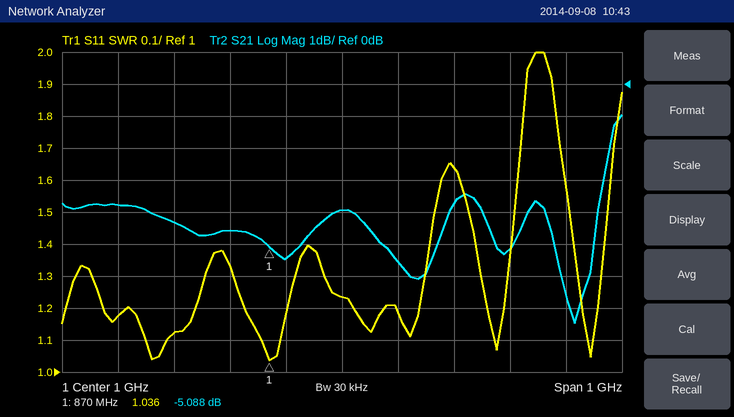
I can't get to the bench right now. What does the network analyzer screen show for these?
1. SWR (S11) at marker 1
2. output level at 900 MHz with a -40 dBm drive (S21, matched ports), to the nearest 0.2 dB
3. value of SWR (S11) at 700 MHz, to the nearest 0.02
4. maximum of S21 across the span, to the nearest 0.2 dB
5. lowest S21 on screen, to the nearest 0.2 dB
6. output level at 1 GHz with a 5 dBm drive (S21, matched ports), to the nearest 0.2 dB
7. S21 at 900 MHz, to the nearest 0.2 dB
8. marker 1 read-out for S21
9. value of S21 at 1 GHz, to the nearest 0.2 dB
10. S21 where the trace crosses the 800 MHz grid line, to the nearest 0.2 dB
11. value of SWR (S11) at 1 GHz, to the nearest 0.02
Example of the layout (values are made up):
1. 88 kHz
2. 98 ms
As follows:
1. 1.036
2. -45.4 dBm
3. 1.12
4. -1.0 dB
5. -7.4 dB
6. 1.0 dBm
7. -5.4 dB
8. -5.088 dB
9. -4.0 dB
10. -4.6 dB
11. 1.24
